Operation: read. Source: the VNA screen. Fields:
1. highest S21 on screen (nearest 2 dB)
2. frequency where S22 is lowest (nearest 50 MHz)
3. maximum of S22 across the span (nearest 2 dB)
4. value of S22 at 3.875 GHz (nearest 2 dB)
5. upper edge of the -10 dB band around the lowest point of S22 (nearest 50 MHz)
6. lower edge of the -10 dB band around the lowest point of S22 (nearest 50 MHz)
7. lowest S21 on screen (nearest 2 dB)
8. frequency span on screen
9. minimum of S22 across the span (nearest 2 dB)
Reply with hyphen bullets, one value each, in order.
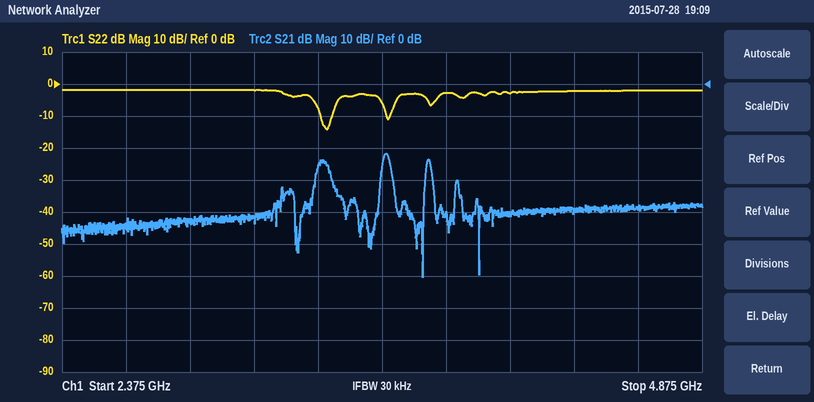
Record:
- -22 dB
- 3.40 GHz
- -2 dB
- -2 dB
- 3.45 GHz
- 3.40 GHz
- -60 dB
- 2.5 GHz
- -14 dB
